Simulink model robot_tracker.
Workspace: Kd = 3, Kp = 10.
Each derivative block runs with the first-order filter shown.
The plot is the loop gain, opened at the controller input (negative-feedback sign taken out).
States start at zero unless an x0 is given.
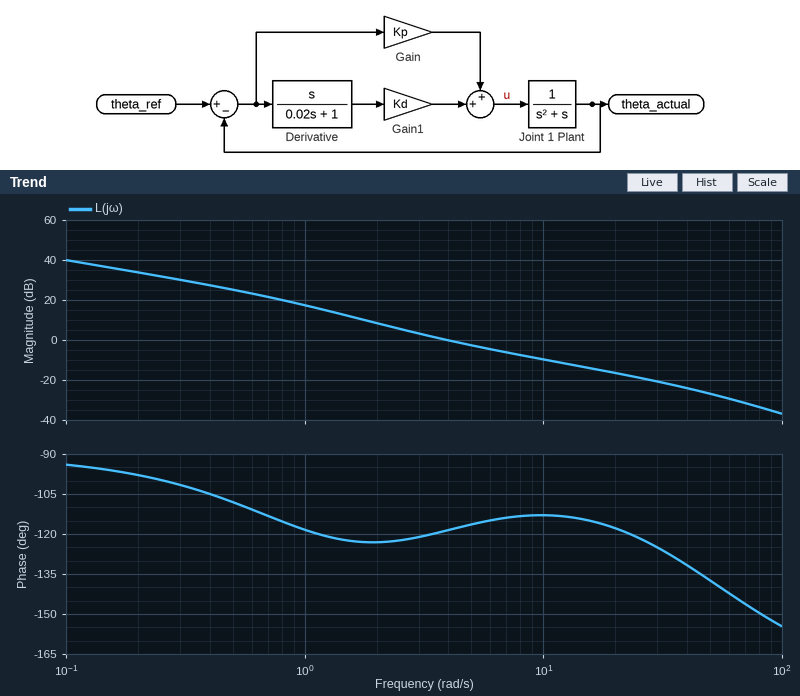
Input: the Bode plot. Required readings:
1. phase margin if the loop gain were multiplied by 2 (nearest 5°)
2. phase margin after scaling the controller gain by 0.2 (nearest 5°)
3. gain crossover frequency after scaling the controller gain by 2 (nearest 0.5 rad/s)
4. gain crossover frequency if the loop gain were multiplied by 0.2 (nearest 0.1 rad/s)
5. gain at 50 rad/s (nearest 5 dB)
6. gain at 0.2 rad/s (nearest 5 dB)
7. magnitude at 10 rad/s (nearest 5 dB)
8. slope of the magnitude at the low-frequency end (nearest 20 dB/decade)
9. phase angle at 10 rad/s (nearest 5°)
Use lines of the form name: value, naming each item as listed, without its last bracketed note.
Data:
phase margin if the loop gain were multiplied by 2: 65°
phase margin after scaling the controller gain by 0.2: 60°
gain crossover frequency after scaling the controller gain by 2: 7.0 rad/s
gain crossover frequency if the loop gain were multiplied by 0.2: 1.3 rad/s
gain at 50 rad/s: -25 dB
gain at 0.2 rad/s: 35 dB
magnitude at 10 rad/s: -10 dB
slope of the magnitude at the low-frequency end: -20 dB/decade
phase angle at 10 rad/s: -115°
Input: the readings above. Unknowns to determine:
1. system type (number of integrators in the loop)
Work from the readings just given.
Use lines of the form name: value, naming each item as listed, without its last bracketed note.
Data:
system type: 1
